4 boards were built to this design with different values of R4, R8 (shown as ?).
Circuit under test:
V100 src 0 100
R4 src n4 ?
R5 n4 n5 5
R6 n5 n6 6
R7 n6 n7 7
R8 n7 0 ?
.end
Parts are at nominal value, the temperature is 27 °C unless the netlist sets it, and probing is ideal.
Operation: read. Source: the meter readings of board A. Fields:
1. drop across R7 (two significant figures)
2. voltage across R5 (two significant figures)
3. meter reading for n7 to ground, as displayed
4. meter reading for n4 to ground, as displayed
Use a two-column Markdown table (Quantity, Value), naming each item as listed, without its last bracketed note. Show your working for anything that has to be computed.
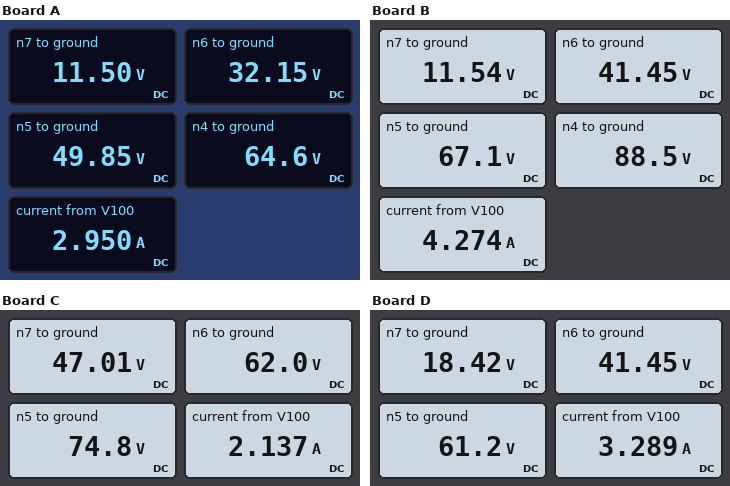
| Quantity | Value |
|---|---|
| drop across R7 | 32.15 V - 11.5 V = 21 V |
| voltage across R5 | 64.6 V - 49.85 V = 15 V |
| meter reading for n7 to ground, as displayed | 11.50 V |
| meter reading for n4 to ground, as displayed | 64.6 V |
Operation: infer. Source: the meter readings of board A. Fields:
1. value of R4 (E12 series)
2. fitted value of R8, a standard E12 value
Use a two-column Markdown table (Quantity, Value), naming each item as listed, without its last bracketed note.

| Quantity | Value |
|---|---|
| value of R4 | 12 Ω |
| fitted value of R8, a standard E12 value | 3.9 Ω |
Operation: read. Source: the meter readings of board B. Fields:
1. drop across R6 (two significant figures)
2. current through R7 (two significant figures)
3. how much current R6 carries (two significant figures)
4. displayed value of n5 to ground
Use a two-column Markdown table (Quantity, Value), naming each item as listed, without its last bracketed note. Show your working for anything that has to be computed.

| Quantity | Value |
|---|---|
| drop across R6 | 67.1 V - 41.45 V = 26 V |
| current through R7 | (41.45 V - 11.54 V) / 7 Ω = 4.3 A |
| how much current R6 carries | (67.1 V - 41.45 V) / 6 Ω = 4.3 A |
| displayed value of n5 to ground | 67.1 V |
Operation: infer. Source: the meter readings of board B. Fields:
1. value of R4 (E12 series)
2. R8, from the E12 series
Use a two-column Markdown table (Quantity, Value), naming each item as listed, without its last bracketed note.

| Quantity | Value |
|---|---|
| value of R4 | 2.7 Ω |
| R8, from the E12 series | 2.7 Ω |
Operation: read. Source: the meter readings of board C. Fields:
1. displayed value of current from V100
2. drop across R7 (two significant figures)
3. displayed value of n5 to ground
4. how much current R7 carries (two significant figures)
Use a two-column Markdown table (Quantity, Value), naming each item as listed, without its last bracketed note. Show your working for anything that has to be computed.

| Quantity | Value |
|---|---|
| displayed value of current from V100 | 2.137 A |
| drop across R7 | 62 V - 47.01 V = 15 V |
| displayed value of n5 to ground | 74.8 V |
| how much current R7 carries | (62 V - 47.01 V) / 7 Ω = 2.1 A |
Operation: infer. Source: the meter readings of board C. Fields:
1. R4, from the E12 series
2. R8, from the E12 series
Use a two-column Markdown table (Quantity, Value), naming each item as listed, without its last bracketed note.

| Quantity | Value |
|---|---|
| R4, from the E12 series | 6.8 Ω |
| R8, from the E12 series | 22 Ω |
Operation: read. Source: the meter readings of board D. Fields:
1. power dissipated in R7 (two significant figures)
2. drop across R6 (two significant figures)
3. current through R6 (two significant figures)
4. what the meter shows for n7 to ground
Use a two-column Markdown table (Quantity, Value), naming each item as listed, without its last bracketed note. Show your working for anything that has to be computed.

| Quantity | Value |
|---|---|
| power dissipated in R7 | (41.45 V - 18.42 V)^2 / 7 Ω = 76 W |
| drop across R6 | 61.2 V - 41.45 V = 20 V |
| current through R6 | (61.2 V - 41.45 V) / 6 Ω = 3.3 A |
| what the meter shows for n7 to ground | 18.42 V |
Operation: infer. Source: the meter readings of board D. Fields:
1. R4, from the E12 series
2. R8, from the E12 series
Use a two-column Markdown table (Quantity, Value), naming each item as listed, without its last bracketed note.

| Quantity | Value |
|---|---|
| R4, from the E12 series | 6.8 Ω |
| R8, from the E12 series | 5.6 Ω |
